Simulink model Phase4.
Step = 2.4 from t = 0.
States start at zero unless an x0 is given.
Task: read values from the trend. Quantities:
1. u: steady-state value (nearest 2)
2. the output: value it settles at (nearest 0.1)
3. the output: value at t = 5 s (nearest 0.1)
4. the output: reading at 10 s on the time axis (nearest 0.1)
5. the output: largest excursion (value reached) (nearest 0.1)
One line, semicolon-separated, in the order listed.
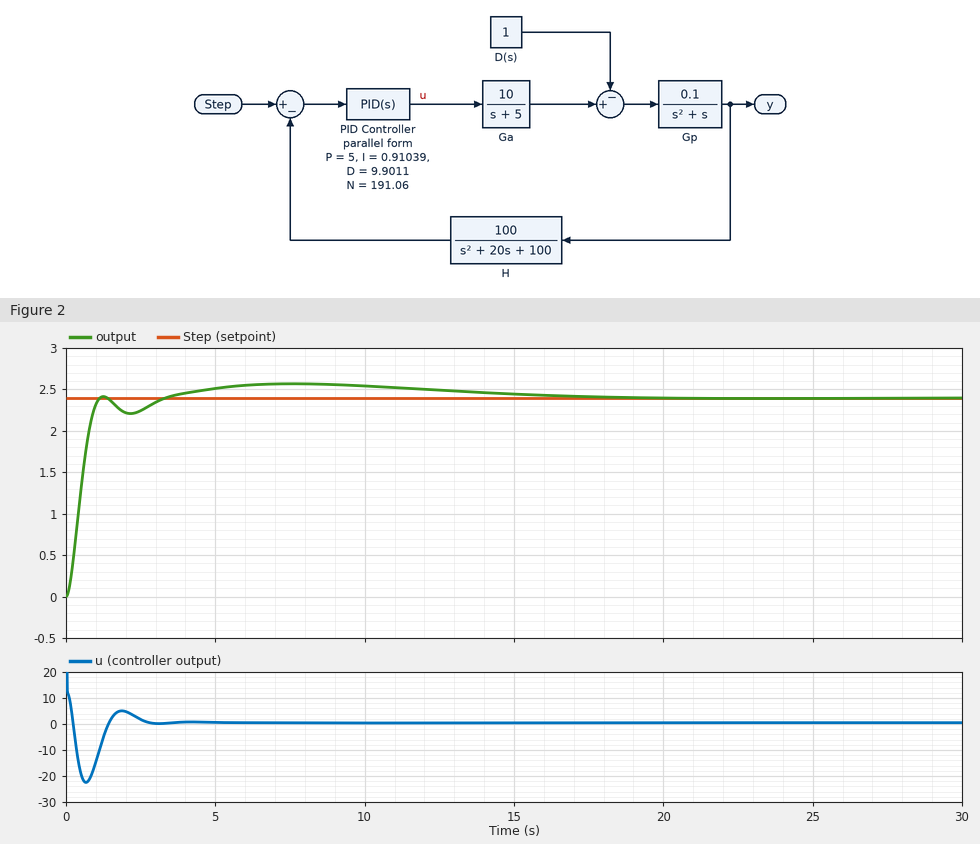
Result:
0; 2.4; 2.5; 2.5; 2.6
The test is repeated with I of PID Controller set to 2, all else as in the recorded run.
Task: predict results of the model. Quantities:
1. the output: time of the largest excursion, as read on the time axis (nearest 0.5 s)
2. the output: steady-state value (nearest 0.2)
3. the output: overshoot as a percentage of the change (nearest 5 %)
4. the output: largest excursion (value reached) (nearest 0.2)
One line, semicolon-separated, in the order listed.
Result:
5.5 s; 2.4; 15 %; 2.8
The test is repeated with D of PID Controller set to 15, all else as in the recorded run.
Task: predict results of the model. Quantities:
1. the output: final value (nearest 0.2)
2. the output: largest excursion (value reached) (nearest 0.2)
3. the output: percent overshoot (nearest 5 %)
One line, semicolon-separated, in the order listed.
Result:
2.4; 2.8; 15 %
